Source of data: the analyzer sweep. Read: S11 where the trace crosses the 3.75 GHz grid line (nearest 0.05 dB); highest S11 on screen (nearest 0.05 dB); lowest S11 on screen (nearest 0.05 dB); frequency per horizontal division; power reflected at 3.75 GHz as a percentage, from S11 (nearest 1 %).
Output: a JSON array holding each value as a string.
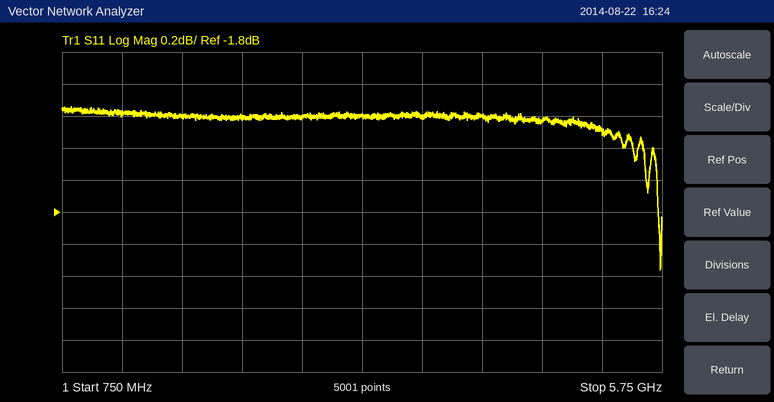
["-1.20 dB", "-1.15 dB", "-2.15 dB", "500 MHz", "76 %"]
